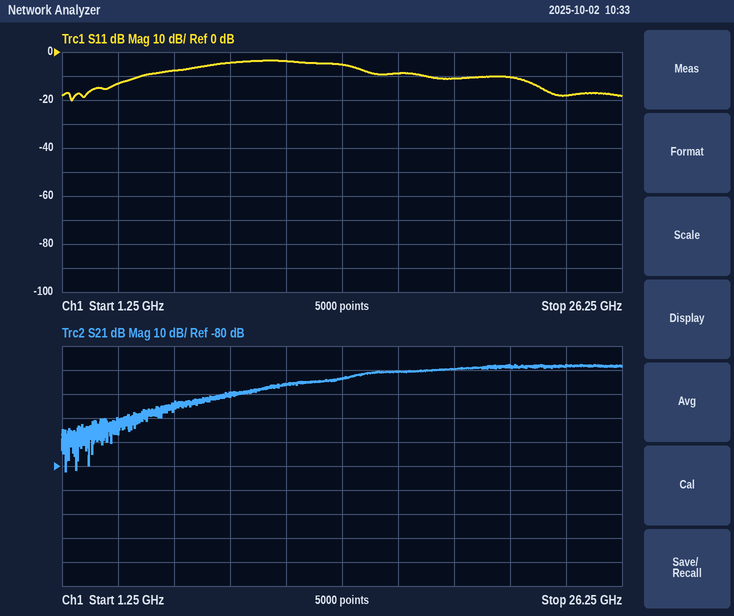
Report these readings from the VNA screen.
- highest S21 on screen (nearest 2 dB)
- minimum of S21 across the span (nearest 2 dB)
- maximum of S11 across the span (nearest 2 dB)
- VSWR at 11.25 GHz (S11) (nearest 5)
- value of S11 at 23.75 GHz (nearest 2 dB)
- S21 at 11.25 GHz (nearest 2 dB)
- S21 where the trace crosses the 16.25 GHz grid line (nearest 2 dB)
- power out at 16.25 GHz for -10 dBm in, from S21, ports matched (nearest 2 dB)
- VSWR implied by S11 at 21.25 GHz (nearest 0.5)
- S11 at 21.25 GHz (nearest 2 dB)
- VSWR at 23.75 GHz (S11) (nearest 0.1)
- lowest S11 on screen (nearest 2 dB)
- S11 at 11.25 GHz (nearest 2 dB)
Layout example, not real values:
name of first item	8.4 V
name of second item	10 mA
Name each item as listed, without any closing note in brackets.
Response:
highest S21 on screen	-38 dB
minimum of S21 across the span	-82 dB
maximum of S11 across the span	-4 dB
VSWR at 11.25 GHz (S11)	5
value of S11 at 23.75 GHz	-18 dB
S21 at 11.25 GHz	-46 dB
S21 where the trace crosses the 16.25 GHz grid line	-40 dB
power out at 16.25 GHz for -10 dBm in, from S21, ports matched	-50 dBm
VSWR implied by S11 at 21.25 GHz	2.0
S11 at 21.25 GHz	-10 dB
VSWR at 23.75 GHz (S11)	1.3
lowest S11 on screen	-20 dB
S11 at 11.25 GHz	-4 dB
